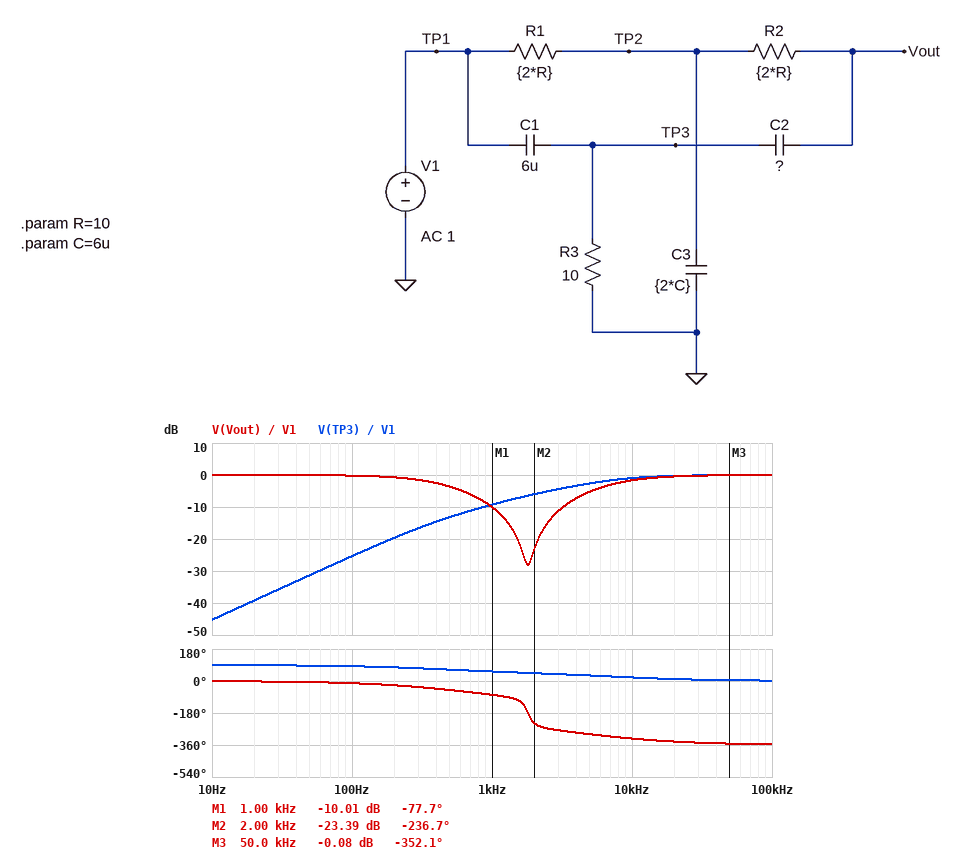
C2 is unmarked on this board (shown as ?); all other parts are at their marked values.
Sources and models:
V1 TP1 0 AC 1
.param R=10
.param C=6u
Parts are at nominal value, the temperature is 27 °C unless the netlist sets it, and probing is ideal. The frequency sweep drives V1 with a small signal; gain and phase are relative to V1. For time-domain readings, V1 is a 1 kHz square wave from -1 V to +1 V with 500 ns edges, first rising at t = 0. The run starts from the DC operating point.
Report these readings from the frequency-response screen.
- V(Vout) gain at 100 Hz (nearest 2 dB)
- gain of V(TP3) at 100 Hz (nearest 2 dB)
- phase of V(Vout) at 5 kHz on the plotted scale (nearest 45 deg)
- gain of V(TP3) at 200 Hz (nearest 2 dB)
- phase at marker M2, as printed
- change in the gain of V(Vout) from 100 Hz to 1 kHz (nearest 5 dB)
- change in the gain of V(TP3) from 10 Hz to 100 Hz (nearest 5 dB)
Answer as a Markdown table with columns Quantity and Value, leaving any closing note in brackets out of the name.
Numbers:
| Quantity | Value |
|---|---|
| V(Vout) gain at 100 Hz | 0 dB |
| gain of V(TP3) at 100 Hz | -26 dB |
| phase of V(Vout) at 5 kHz on the plotted scale | -315 deg |
| gain of V(TP3) at 200 Hz | -20 dB |
| phase at marker M2, as printed | -236.7 deg |
| change in the gain of V(Vout) from 100 Hz to 1 kHz | -10 dB |
| change in the gain of V(TP3) from 10 Hz to 100 Hz | 20 dB |
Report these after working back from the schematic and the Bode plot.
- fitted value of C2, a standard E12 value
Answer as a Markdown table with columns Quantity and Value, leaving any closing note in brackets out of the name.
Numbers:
| Quantity | Value |
|---|---|
| fitted value of C2, a standard E12 value | 2.7 µF |
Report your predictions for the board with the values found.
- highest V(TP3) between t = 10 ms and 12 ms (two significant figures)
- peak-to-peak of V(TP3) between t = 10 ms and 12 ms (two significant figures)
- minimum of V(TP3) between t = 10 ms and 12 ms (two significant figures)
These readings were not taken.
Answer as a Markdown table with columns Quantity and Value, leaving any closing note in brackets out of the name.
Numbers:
| Quantity | Value |
|---|---|
| highest V(TP3) between t = 10 ms and 12 ms | 1.9 V |
| peak-to-peak of V(TP3) between t = 10 ms and 12 ms | 3.9 V |
| minimum of V(TP3) between t = 10 ms and 12 ms | -1.9 V |
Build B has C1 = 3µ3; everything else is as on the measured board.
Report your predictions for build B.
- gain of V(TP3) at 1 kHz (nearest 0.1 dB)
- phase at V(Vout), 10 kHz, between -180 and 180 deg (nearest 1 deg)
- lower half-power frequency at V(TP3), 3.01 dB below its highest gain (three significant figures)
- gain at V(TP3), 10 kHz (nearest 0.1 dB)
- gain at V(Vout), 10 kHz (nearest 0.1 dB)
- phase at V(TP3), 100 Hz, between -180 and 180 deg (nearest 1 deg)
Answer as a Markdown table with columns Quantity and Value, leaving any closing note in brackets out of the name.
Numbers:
| Quantity | Value |
|---|---|
| gain of V(TP3) at 1 kHz | -13.4 dB |
| phase at V(Vout), 10 kHz, between -180 and 180 deg | 49 deg |
| lower half-power frequency at V(TP3), 3.01 dB below its highest gain | 8.18 kHz |
| gain at V(TP3), 10 kHz | -2.3 dB |
| gain at V(Vout), 10 kHz | -3.0 dB |
| phase at V(TP3), 100 Hz, between -180 and 180 deg | 82 deg |
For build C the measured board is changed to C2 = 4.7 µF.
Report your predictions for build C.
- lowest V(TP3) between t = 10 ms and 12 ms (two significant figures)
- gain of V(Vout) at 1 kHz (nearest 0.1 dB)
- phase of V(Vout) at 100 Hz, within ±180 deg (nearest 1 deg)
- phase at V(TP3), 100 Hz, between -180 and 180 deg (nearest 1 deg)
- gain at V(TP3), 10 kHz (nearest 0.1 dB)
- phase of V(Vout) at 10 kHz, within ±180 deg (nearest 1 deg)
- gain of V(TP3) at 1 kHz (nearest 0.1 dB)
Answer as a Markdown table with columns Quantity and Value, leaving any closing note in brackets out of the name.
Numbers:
| Quantity | Value |
|---|---|
| lowest V(TP3) between t = 10 ms and 12 ms | -1.9 V |
| gain of V(Vout) at 1 kHz | -14.2 dB |
| phase of V(Vout) at 100 Hz, within ±180 deg | -15 deg |
| phase at V(TP3), 100 Hz, between -180 and 180 deg | 80 deg |
| gain at V(TP3), 10 kHz | -0.9 dB |
| phase of V(Vout) at 10 kHz, within ±180 deg | 30 deg |
| gain of V(TP3) at 1 kHz | -9.8 dB |
